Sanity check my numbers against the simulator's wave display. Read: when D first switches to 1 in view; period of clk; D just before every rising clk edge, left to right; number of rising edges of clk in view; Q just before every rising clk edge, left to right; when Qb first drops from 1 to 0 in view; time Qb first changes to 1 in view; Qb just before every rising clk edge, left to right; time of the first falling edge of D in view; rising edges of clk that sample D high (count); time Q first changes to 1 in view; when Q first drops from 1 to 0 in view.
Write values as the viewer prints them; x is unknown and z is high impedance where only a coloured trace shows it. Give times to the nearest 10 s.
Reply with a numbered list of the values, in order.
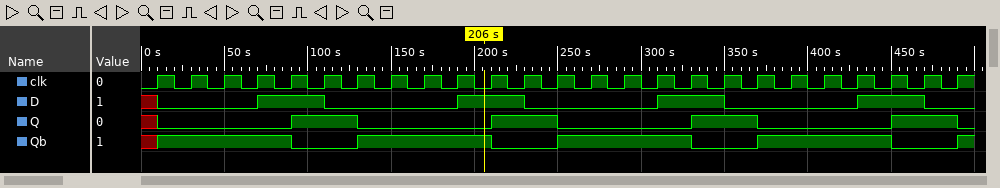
1. 70 s
2. 20 s
3. x 0 0 0 1 1 0 0 0 0 1 1 0 0 0 0 1 1 0 0 0 0 1 1 0
4. 25
5. x 0 0 0 0 1 1 0 0 0 0 1 1 0 0 0 0 1 1 0 0 0 0 1 1
6. 90 s
7. 10 s
8. x 1 1 1 1 0 0 1 1 1 1 0 0 1 1 1 1 0 0 1 1 1 1 0 0
9. 110 s
10. 8
11. 90 s
12. 130 s
